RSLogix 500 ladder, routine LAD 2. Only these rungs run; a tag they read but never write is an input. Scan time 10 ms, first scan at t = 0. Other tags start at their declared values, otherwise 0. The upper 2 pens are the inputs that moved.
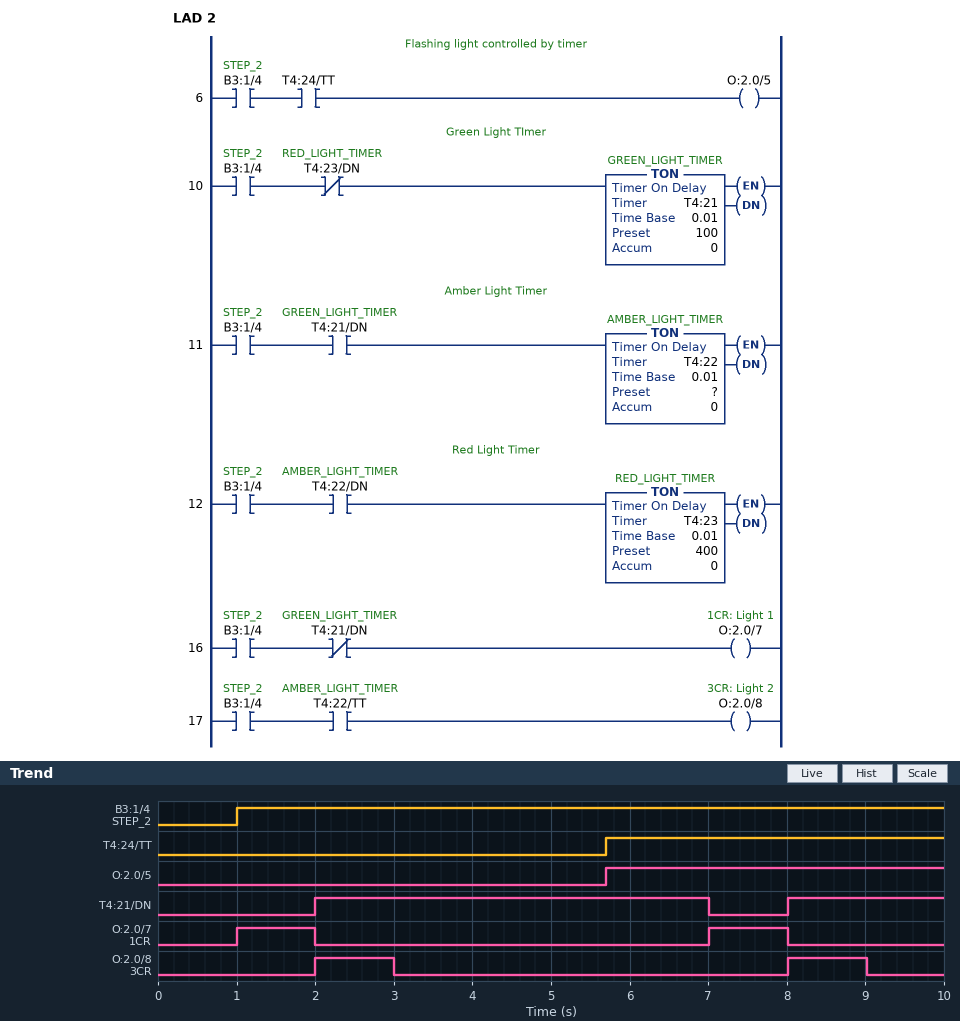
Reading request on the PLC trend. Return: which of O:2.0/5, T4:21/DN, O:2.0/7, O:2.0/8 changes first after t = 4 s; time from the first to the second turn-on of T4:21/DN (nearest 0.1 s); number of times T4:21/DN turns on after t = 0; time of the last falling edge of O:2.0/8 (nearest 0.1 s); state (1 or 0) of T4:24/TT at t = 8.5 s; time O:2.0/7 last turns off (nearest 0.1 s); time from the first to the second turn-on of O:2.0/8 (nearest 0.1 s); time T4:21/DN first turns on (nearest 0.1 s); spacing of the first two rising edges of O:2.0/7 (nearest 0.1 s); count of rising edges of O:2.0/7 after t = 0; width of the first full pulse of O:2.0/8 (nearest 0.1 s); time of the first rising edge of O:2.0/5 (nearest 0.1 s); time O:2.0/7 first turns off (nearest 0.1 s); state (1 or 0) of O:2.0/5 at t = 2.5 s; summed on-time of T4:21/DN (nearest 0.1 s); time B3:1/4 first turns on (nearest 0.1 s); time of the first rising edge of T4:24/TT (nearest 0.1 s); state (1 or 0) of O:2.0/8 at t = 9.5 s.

O:2.0/5
6.0 s
2
9.0 s
1
8.0 s
6.0 s
2.0 s
6.0 s
2
1.0 s
5.7 s
2.0 s
0
7.0 s
1.0 s
5.7 s
0
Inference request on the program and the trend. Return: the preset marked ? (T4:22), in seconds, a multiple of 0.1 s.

1.0 s
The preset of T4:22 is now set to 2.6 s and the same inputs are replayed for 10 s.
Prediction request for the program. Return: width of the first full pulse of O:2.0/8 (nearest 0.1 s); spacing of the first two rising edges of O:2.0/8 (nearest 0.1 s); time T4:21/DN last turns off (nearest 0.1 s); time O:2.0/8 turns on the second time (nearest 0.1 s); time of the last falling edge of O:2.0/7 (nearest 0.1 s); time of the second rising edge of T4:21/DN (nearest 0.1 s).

2.6 s
7.6 s
8.6 s
9.6 s
9.6 s
9.6 s
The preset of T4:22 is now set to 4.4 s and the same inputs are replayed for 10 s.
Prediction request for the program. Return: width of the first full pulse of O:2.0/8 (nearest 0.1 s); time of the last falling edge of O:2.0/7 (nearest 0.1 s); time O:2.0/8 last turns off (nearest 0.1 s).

4.4 s
2.0 s
6.4 s
